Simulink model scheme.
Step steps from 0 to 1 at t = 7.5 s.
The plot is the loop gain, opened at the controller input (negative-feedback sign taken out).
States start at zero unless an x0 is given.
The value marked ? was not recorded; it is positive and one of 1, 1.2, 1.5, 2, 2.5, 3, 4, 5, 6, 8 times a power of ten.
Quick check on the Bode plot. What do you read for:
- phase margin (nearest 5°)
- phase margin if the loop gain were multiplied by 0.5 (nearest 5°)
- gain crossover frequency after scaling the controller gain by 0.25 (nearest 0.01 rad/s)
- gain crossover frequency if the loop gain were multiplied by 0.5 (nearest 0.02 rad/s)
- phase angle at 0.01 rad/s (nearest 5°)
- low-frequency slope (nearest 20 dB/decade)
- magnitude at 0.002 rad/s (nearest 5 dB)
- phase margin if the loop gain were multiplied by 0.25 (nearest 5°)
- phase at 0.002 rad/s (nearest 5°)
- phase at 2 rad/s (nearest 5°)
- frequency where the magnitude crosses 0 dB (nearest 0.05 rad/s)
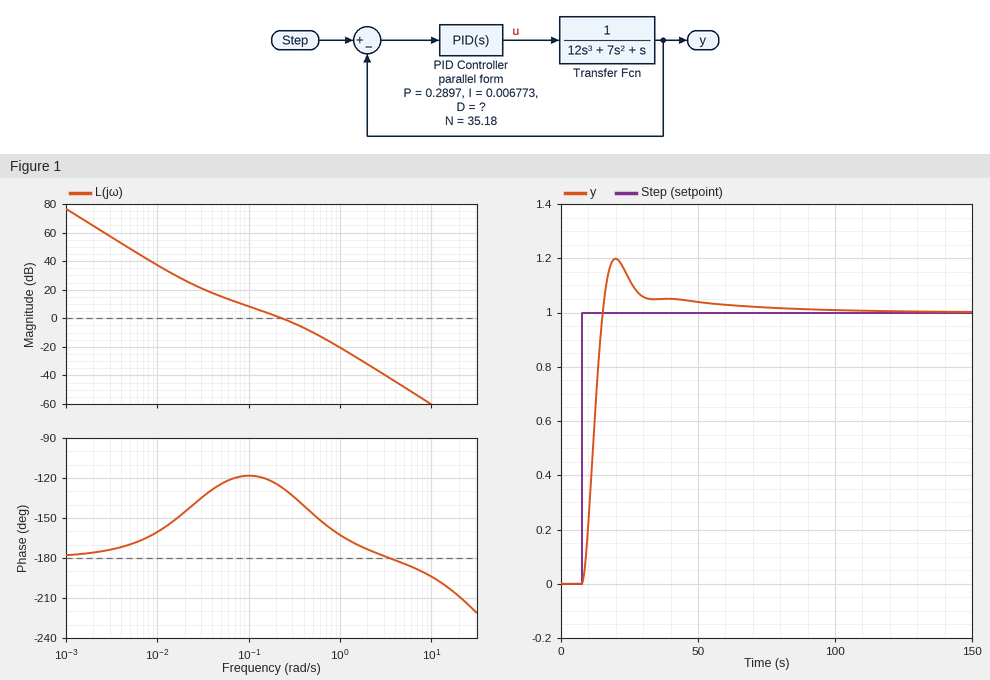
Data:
55°
60°
0.07 rad/s
0.12 rad/s
-160°
-40 dB/decade
65 dB
60°
-175°
-175°
0.25 rad/s
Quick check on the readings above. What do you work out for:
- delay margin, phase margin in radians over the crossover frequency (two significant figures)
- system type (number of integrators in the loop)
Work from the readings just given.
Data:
3.8 s
2
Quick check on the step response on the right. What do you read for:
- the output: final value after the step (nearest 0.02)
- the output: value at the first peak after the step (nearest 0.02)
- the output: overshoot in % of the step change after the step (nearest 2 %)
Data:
1.00
1.20
20 %
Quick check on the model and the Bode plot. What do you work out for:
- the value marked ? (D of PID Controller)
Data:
1.2
